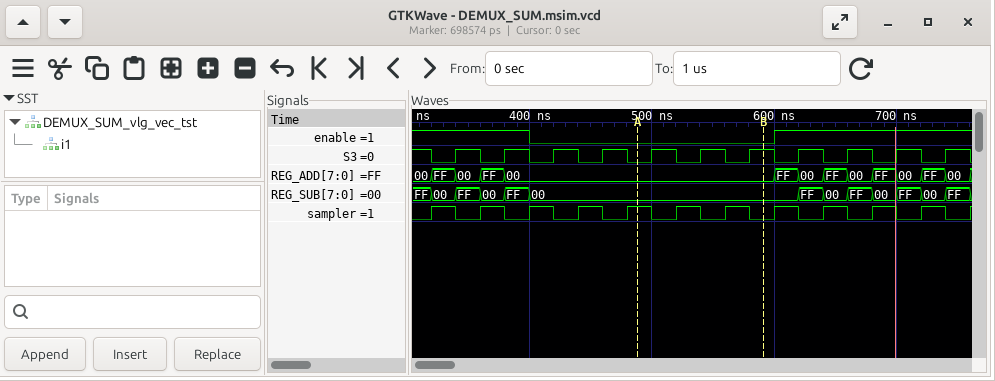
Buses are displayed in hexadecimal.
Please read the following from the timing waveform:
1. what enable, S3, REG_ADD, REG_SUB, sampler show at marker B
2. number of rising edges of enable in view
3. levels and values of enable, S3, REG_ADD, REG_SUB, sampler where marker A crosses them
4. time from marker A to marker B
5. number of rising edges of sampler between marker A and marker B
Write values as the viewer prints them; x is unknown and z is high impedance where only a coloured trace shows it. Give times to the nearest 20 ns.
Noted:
enable=0, S3=1, REG_ADD=00, REG_SUB=00, sampler=0
1
enable=0, S3=0, REG_ADD=00, REG_SUB=00, sampler=1
100 ns
2
